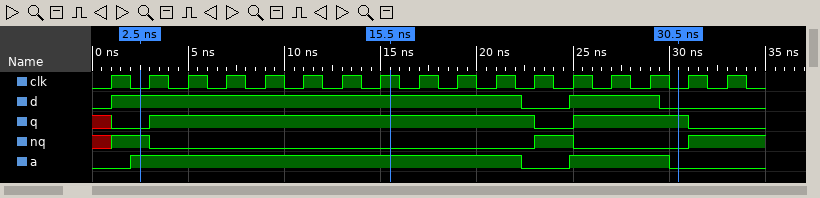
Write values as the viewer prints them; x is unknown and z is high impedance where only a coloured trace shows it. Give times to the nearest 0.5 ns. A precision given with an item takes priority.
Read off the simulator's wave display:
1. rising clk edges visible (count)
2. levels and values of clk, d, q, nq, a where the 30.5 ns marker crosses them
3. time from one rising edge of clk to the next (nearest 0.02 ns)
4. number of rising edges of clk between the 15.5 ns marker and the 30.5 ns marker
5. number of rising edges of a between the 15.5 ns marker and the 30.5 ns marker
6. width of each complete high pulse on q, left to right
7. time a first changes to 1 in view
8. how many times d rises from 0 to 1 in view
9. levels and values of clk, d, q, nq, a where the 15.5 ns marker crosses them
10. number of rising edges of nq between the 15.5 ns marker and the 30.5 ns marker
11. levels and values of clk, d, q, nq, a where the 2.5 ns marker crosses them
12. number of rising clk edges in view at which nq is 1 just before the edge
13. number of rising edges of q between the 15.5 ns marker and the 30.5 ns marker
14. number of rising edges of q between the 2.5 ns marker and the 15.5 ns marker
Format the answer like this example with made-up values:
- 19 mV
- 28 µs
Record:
- 17
- clk=0, d=0, q=1, nq=0, a=0
- 2 ns
- 7
- 1
- 20 ns, 6 ns
- 2 ns
- 2
- clk=1, d=1, q=1, nq=0, a=1
- 1
- clk=0, d=1, q=0, nq=1, a=1
- 3
- 1
- 1
